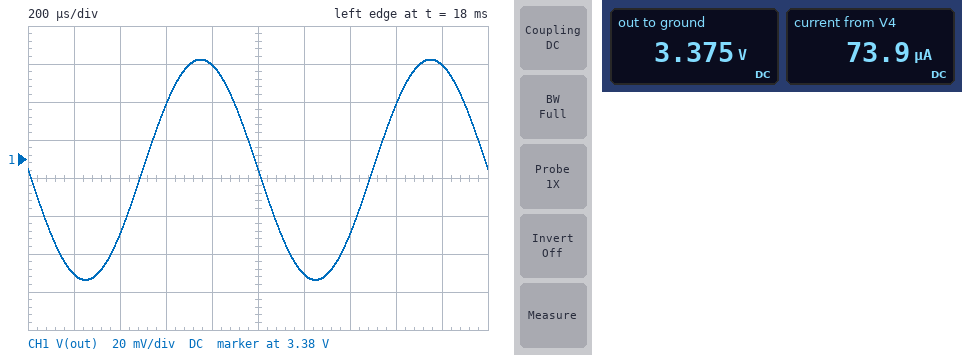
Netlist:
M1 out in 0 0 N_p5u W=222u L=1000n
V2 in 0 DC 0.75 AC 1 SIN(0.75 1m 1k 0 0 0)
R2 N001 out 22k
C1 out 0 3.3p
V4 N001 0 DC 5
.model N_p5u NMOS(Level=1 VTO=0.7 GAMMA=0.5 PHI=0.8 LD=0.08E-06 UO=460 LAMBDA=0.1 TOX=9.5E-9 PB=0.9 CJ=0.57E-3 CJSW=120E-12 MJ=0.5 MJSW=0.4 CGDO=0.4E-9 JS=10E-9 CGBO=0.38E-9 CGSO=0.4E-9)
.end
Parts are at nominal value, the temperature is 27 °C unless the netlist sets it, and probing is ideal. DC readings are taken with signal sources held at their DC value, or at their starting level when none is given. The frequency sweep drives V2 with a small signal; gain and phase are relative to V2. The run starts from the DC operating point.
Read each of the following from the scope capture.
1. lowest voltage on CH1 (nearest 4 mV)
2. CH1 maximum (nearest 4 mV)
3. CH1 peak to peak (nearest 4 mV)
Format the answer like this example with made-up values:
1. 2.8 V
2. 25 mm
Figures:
1. 3.316 V
2. 3.432 V
3. 116 mV
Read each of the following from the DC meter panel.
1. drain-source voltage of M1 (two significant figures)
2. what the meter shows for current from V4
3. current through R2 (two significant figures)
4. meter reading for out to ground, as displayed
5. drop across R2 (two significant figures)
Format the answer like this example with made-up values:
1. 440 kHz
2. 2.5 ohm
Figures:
1. 3.4 V
2. 73.9 µA
3. 74 µA
4. 3.375 V
5. 1.6 V
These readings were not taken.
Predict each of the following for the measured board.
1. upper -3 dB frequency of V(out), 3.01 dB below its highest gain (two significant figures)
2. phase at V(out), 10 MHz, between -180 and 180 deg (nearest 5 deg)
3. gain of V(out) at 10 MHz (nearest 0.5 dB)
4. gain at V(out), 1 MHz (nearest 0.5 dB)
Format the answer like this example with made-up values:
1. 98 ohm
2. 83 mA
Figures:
1. 2.4 MHz
2. 105 deg
3. 22.5 dB
4. 34.5 dB
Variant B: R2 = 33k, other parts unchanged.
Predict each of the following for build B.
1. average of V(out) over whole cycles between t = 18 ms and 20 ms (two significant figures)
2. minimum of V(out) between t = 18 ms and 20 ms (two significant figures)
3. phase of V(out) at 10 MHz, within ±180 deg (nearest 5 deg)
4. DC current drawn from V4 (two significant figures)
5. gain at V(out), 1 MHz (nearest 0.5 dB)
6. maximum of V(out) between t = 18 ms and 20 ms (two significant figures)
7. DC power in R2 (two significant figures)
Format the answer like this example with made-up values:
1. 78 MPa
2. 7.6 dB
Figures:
1. 2.7 V
2. 2.6 V
3. 100 deg
4. 70 µA
5. 36.5 dB
6. 2.8 V
7. 160 µW
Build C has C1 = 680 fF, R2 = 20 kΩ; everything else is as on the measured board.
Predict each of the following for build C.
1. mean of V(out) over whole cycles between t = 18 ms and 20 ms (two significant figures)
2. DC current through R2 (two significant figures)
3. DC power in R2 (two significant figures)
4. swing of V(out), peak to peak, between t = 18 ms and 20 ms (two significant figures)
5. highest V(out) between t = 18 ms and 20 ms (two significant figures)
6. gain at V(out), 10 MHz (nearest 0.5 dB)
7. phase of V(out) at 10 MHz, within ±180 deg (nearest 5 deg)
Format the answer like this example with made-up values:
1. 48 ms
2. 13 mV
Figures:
1. 3.5 V
2. 75 µA
3. 110 µW
4. 110 mV
5. 3.6 V
6. 32.0 dB
7. 140 deg
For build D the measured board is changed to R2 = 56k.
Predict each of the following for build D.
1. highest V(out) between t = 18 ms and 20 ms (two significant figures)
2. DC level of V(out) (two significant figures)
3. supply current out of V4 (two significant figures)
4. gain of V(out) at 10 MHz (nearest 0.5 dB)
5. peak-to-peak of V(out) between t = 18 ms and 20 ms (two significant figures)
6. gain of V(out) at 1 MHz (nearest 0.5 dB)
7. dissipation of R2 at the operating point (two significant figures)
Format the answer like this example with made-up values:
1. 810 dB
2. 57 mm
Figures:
1. 1.6 V
2. 1.5 V
3. 63 µA
4. 21.5 dB
5. 220 mV
6. 38.0 dB
7. 220 µW
